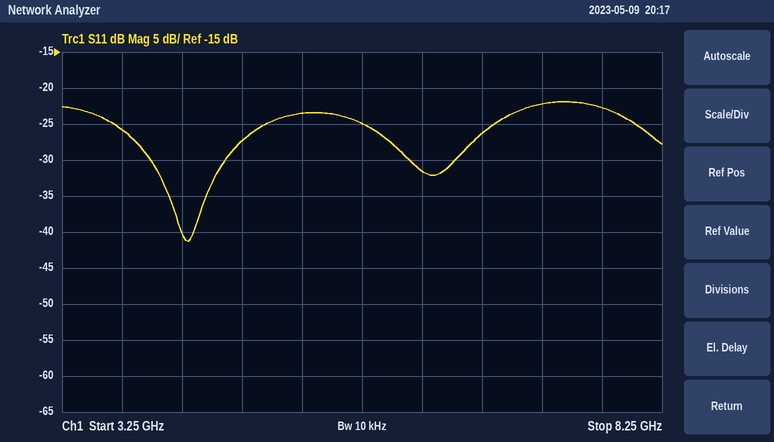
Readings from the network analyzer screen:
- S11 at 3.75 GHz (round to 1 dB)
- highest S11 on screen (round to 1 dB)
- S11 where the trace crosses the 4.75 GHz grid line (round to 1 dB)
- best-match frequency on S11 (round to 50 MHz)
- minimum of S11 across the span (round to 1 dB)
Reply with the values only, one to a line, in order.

-26 dB
-22 dB
-27 dB
4.30 GHz
-41 dB
